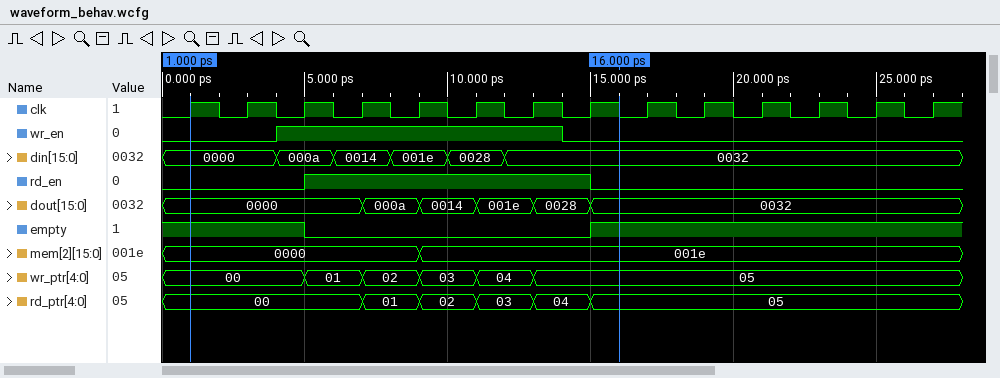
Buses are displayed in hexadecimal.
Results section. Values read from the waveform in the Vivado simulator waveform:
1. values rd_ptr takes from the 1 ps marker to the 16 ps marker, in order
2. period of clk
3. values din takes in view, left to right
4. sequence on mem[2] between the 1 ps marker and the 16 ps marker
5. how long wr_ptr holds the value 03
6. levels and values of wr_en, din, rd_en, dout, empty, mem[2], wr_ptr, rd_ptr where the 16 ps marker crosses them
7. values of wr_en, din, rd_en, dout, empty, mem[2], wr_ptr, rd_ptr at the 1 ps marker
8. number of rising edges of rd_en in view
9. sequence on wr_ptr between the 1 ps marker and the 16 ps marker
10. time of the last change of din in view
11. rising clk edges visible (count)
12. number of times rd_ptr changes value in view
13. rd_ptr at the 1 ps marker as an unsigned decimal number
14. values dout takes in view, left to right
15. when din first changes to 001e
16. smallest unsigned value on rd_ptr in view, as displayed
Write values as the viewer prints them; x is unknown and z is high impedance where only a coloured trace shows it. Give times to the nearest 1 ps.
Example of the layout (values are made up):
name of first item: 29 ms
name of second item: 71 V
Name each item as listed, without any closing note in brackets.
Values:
values rd_ptr takes from the 1 ps marker to the 16 ps marker, in order: 00, 01, 02, 03, 04, 05
period of clk: 2 ps
values din takes in view, left to right: 0000, 000a, 0014, 001e, 0028, 0032
sequence on mem[2] between the 1 ps marker and the 16 ps marker: 0000, 001e
how long wr_ptr holds the value 03: 2 ps
levels and values of wr_en, din, rd_en, dout, empty, mem[2], wr_ptr, rd_ptr where the 16 ps marker crosses them: wr_en=0, din=0032, rd_en=0, dout=0032, empty=1, mem[2]=001e, wr_ptr=05, rd_ptr=05
values of wr_en, din, rd_en, dout, empty, mem[2], wr_ptr, rd_ptr at the 1 ps marker: wr_en=0, din=0000, rd_en=0, dout=0000, empty=1, mem[2]=0000, wr_ptr=00, rd_ptr=00
number of rising edges of rd_en in view: 1
sequence on wr_ptr between the 1 ps marker and the 16 ps marker: 00, 01, 02, 03, 04, 05
time of the last change of din in view: 12 ps
rising clk edges visible: 14
number of times rd_ptr changes value in view: 5
rd_ptr at the 1 ps marker as an unsigned decimal number: 0
values dout takes in view, left to right: 0000, 000a, 0014, 001e, 0028, 0032
when din first changes to 001e: 8 ps
smallest unsigned value on rd_ptr in view, as displayed: 00
